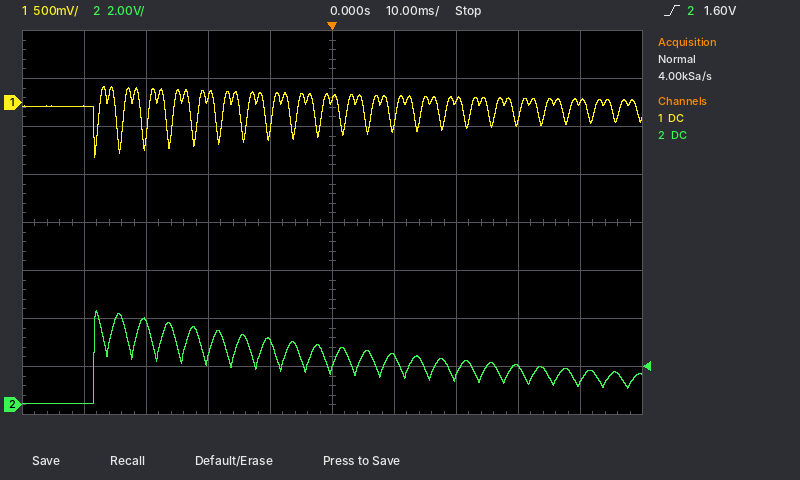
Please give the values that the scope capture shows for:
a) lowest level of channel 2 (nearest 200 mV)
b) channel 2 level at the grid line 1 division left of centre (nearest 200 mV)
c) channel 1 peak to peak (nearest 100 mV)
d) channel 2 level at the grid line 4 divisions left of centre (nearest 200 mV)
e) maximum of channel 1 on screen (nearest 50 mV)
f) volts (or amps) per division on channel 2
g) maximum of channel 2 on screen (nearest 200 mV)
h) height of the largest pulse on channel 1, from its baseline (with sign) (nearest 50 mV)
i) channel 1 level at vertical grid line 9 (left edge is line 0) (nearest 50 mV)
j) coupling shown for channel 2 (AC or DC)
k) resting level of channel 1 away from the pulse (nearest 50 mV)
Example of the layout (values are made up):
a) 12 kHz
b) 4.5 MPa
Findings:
a) 0.0 V
b) 2.6 V
c) 700 mV
d) 0.0 V
e) 150 mV
f) 2 V
g) 4.0 V
h) -550 mV
i) 0 mV
j) DC
k) 0 mV
